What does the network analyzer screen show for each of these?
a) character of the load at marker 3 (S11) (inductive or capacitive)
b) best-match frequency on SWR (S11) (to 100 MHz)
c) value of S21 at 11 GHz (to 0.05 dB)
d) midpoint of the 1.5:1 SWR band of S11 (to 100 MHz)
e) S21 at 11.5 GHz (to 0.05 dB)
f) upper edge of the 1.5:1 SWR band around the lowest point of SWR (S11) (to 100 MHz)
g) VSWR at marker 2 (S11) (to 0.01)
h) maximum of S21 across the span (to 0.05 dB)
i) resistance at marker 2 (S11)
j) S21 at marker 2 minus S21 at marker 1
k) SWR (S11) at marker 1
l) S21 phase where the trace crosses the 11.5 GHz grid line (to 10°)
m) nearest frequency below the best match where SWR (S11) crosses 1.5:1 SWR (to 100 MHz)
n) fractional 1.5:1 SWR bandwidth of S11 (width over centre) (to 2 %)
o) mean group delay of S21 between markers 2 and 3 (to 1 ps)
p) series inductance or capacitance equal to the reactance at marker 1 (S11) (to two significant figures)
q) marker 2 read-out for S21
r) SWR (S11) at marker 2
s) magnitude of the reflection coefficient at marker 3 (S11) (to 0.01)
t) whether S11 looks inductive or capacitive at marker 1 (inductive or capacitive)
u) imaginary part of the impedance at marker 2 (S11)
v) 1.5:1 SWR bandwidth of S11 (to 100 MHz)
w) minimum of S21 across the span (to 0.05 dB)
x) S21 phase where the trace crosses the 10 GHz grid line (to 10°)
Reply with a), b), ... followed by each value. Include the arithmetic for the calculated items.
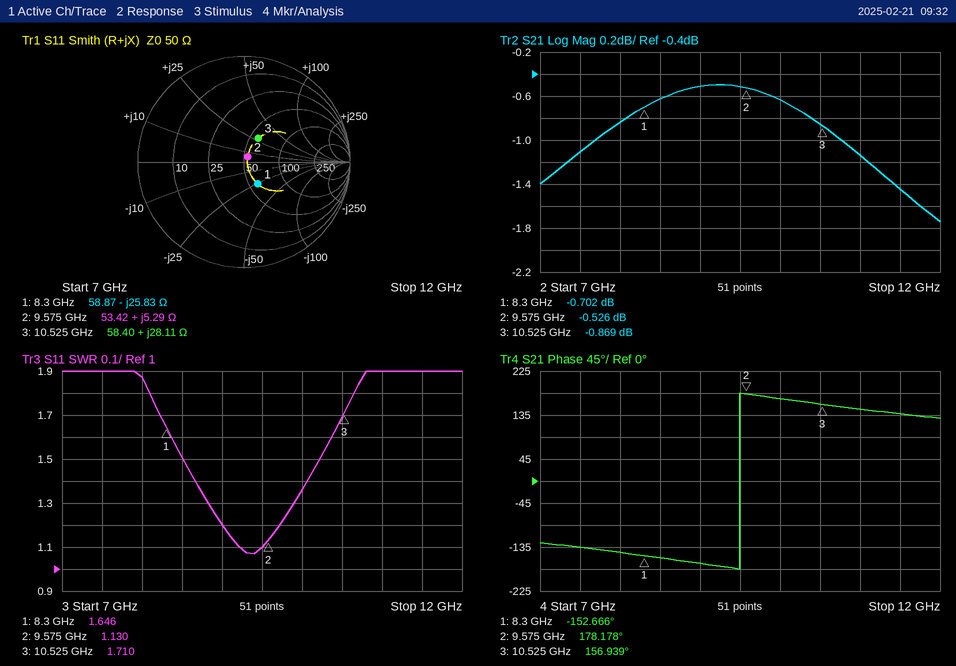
a) inductive
b) 9.4 GHz
c) -1.15 dB
d) 9.4 GHz
e) -1.45 dB
f) 10.2 GHz
g) 1.13
h) -0.50 dB
i) 53.42 Ω
j) -0.526 − (-0.702) = 0.176 dB
k) 1.646
l) 140°
m) 8.5 GHz
n) 1.7 GHz / 9.35 GHz ≈ 18 %
o) −(156.939° − (178.178°))/(360° × 950 MHz) ≈ 62 ps
p) C = 1/(2π × 8.3 GHz × 25.83 Ω) ≈ 742 fF, so 740 fF to two significant figures
q) -0.526 dB
r) 1.130
s) 0.26
t) capacitive
u) +5.29 Ω
v) 10.2 GHz − 8.5 GHz = 1.7 GHz
w) -1.75 dB
x) 170°
